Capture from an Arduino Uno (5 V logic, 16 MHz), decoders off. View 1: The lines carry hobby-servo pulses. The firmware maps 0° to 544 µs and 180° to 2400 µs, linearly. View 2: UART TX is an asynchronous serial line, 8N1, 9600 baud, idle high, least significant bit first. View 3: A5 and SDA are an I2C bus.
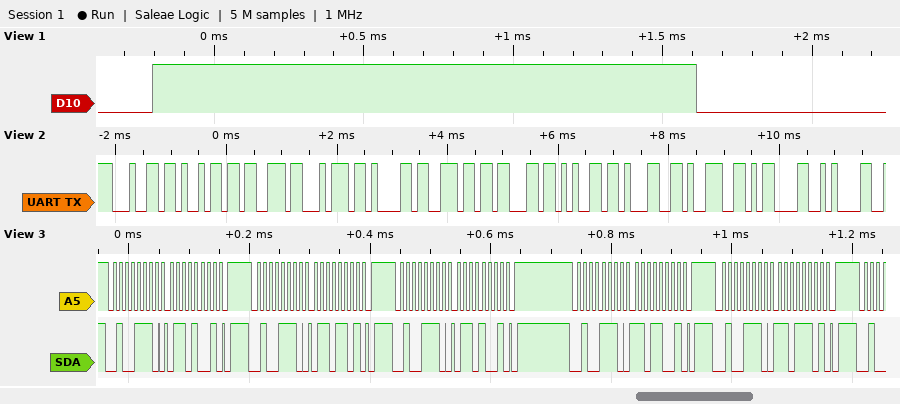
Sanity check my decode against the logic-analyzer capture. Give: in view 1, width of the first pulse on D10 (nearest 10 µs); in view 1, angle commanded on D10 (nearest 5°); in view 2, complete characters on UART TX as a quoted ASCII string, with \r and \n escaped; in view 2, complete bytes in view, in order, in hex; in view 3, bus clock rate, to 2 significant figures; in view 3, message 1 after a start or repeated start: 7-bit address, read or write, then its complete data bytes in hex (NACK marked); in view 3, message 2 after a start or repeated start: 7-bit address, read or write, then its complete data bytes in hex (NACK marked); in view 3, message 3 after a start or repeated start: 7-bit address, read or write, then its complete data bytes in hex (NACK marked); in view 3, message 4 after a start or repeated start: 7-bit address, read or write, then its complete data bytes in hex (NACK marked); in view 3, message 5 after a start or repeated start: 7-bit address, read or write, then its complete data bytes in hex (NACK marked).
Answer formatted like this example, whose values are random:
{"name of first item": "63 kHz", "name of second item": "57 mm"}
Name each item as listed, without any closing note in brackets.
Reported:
{"in view 1, width of the first pulse on D10": "1820 µs", "in view 1, angle commanded on D10": "125°", "in view 2, complete characters on UART TX as a quoted ASCII string, with \\r and \\n escaped": "\"distance19\\r\\n\"", "in view 2, complete bytes in view, in order, in hex": "64 69 73 74 61 6E 63 65 31 39 0D 0A", "in view 3, bus clock rate, to 2 significant figures": "100 kHz", "in view 3, message 1 after a start or repeated start: 7-bit address, read or write, then its complete data bytes in hex": "0x27 write: 69", "in view 3, message 2 after a start or repeated start: 7-bit address, read or write, then its complete data bytes in hex": "0x27 write: 6D", "in view 3, message 3 after a start or repeated start: 7-bit address, read or write, then its complete data bytes in hex": "0x27 write: 69", "in view 3, message 4 after a start or repeated start: 7-bit address, read or write, then its complete data bytes in hex": "0x27 write: D9", "in view 3, message 5 after a start or repeated start: 7-bit address, read or write, then its complete data bytes in hex": "0x27 write: DD"}
